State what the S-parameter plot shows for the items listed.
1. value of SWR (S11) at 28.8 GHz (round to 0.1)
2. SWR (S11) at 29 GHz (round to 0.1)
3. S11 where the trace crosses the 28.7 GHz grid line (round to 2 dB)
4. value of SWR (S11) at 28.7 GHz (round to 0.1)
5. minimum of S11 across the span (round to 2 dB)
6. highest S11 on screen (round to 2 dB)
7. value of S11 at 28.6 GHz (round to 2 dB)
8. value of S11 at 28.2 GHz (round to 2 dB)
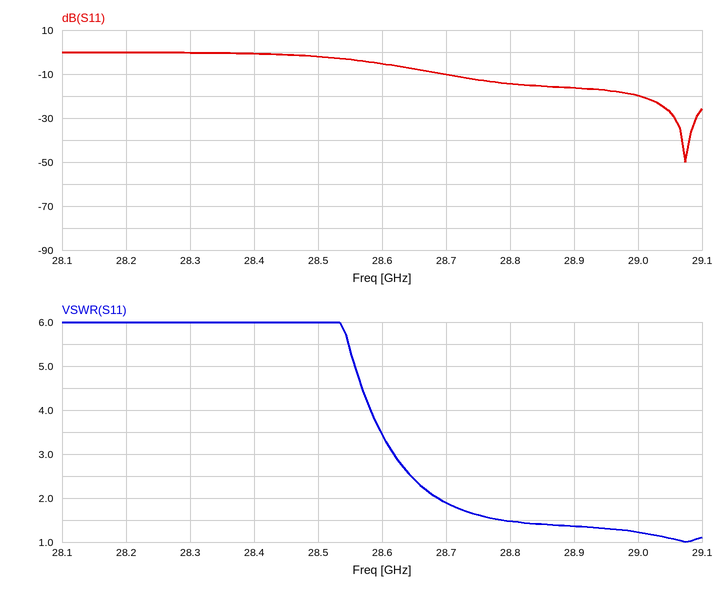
1.5
1.2
-10 dB
1.9
-50 dB
0 dB
-6 dB
0 dB
